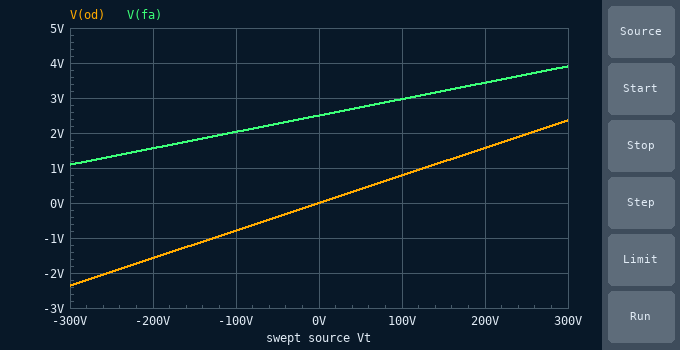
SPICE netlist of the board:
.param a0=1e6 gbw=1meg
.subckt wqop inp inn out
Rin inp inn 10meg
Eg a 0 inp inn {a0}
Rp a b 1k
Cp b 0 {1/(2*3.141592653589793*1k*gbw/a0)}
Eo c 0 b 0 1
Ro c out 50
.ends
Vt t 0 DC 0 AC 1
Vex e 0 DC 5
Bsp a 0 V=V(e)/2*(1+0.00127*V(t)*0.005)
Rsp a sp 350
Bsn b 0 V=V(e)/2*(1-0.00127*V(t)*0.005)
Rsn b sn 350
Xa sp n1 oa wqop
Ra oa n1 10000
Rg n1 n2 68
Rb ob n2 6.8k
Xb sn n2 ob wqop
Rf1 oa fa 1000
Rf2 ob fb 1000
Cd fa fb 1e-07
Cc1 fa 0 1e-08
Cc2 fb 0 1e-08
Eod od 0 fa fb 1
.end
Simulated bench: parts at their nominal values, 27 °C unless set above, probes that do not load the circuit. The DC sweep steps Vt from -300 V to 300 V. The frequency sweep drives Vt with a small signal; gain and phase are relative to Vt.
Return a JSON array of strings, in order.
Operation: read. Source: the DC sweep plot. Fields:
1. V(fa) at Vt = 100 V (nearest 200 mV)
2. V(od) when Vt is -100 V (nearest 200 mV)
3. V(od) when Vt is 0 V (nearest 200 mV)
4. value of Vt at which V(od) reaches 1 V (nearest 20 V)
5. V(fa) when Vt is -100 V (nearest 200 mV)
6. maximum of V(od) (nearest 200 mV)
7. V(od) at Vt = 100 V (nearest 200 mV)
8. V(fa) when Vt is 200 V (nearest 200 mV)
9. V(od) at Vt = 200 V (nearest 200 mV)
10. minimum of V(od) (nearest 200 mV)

["3.0 V", "-800 mV", "0 V", "120 V", "2.0 V", "2.4 V", "800 mV", "3.4 V", "1.6 V", "-2.4 V"]
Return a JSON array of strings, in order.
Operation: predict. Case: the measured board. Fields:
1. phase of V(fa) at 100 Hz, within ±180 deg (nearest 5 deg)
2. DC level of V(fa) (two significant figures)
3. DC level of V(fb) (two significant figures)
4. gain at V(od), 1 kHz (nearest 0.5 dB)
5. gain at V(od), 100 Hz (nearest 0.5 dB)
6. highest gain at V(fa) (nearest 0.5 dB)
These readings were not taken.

["-10 deg", "2.5 V", "2.5 V", "-46.5 dB", "-42.0 dB", "-46.5 dB"]
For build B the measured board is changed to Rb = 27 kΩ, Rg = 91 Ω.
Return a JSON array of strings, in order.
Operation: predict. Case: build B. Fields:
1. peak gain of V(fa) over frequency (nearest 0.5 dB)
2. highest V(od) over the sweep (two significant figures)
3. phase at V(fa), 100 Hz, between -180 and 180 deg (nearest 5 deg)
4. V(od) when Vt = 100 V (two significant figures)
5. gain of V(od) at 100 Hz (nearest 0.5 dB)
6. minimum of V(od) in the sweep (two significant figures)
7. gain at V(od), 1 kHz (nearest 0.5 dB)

["-49.0 dB", "3.9 V", "-15 deg", "1.3 V", "-38.0 dB", "-3.9 V", "-43.0 dB"]
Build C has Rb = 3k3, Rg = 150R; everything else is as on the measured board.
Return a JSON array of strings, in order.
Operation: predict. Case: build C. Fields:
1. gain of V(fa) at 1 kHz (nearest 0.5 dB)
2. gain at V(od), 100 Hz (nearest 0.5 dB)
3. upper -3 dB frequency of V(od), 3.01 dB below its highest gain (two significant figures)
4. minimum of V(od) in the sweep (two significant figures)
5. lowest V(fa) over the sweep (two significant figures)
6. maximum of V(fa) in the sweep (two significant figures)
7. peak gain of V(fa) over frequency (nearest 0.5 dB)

["-57.0 dB", "-51.0 dB", "760 Hz", "-850 mV", "1.9 V", "3.1 V", "-53.5 dB"]
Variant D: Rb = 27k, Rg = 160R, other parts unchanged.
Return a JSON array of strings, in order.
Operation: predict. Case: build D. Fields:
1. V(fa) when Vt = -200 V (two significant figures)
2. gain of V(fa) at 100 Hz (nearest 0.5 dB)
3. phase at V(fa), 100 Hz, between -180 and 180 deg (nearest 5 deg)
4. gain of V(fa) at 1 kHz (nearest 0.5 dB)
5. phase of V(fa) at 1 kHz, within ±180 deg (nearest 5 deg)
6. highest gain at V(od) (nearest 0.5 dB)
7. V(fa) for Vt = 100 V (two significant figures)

["2.1 V", "-54.0 dB", "-15 deg", "-55.5 dB", "-115 deg", "-42.5 dB", "2.7 V"]
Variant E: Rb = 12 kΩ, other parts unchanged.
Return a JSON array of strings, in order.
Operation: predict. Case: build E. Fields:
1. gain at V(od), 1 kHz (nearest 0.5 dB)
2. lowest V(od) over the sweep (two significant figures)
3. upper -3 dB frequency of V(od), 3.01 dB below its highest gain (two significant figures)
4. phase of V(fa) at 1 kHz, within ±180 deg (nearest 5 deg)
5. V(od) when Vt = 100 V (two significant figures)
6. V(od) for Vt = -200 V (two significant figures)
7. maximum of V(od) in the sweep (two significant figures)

["-44.5 dB", "-3.1 V", "720 Hz", "-80 deg", "1.0 V", "-2.1 V", "3.1 V"]
